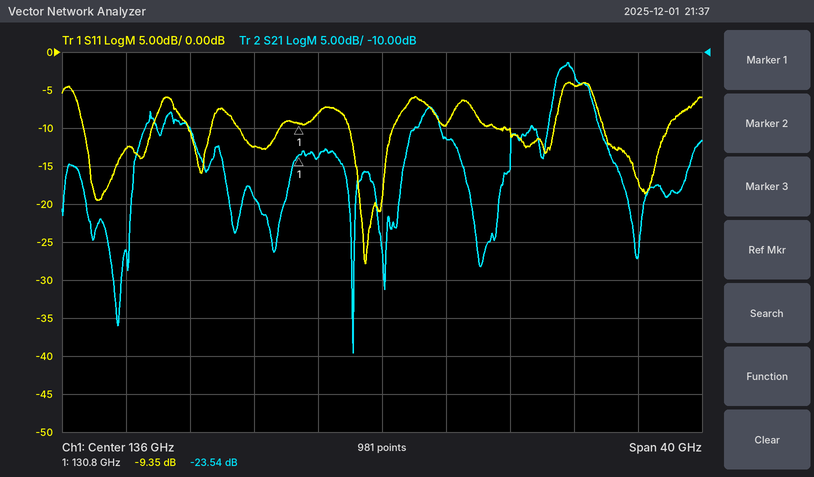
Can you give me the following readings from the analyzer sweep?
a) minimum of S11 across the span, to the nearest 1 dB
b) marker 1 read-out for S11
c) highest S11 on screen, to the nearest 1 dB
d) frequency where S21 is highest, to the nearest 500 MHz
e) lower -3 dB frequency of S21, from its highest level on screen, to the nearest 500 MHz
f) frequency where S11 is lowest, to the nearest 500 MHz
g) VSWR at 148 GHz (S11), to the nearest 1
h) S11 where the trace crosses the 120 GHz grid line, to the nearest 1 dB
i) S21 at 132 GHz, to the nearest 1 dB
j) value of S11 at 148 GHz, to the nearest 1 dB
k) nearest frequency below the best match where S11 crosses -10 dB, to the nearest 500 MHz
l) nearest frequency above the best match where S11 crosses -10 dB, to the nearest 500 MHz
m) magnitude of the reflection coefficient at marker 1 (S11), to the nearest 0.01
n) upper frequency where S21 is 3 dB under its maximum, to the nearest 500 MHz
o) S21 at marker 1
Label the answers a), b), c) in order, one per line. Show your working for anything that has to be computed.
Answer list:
a) -28 dB
b) -9.35 dB
c) -4 dB
d) 147.5 GHz
e) 147.0 GHz
f) 135.0 GHz
g) |Γ| = 10^(-4/20) = 0.6310; VSWR = (1 + 0.6310)/(1 − 0.6310) ≈ 4
h) -13 dB
i) -24 dB
j) -4 dB
k) 134.0 GHz
l) 136.5 GHz
m) 10^(-9.35/20) ≈ 0.34
n) 149.0 GHz
o) -23.54 dB
